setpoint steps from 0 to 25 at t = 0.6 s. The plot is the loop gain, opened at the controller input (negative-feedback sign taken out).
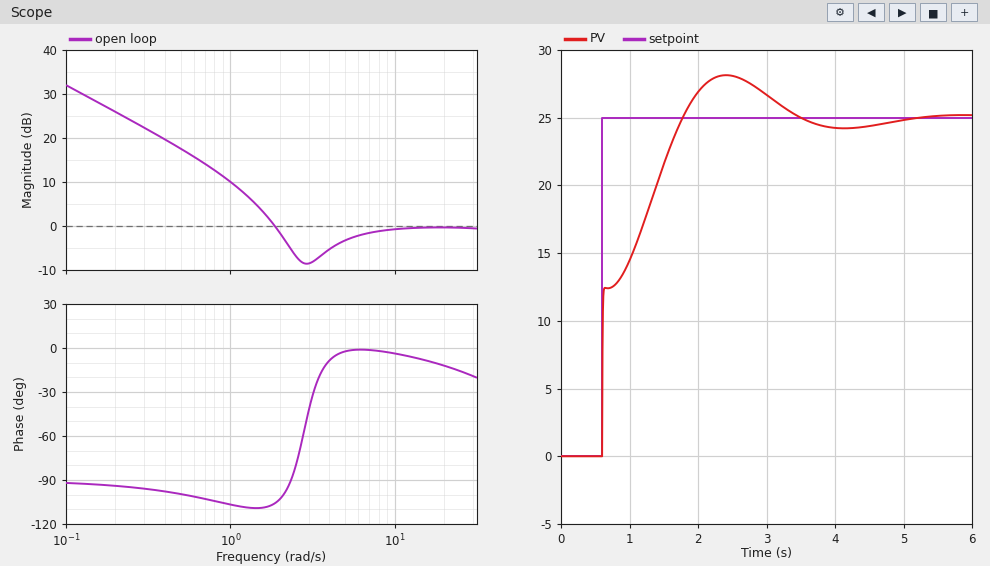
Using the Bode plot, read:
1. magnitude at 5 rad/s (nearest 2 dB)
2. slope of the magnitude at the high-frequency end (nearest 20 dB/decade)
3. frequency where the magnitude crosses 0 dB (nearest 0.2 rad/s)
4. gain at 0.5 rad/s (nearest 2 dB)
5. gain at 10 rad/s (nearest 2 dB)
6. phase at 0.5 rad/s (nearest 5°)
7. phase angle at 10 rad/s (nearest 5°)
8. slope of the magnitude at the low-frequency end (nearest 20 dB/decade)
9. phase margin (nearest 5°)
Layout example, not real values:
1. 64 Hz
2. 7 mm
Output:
1. -4 dB
2. 0 dB/decade
3. 1.8 rad/s
4. 18 dB
5. 0 dB
6. -100°
7. -5°
8. -20 dB/decade
9. 75°
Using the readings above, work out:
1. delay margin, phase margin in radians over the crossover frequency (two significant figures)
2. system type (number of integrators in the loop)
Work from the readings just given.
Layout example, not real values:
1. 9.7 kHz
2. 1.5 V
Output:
1. 0.73 s
2. 1
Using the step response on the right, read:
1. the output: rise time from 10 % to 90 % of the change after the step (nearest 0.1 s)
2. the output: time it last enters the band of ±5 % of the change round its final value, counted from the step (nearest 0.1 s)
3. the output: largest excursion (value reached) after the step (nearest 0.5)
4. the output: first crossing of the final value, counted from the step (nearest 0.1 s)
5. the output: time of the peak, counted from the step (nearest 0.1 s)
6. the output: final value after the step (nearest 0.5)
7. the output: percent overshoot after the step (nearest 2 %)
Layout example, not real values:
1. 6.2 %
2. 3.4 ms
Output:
1. 1.0 s
2. 2.5 s
3. 28.0
4. 1.2 s
5. 1.8 s
6. 25.0
7. 12 %
